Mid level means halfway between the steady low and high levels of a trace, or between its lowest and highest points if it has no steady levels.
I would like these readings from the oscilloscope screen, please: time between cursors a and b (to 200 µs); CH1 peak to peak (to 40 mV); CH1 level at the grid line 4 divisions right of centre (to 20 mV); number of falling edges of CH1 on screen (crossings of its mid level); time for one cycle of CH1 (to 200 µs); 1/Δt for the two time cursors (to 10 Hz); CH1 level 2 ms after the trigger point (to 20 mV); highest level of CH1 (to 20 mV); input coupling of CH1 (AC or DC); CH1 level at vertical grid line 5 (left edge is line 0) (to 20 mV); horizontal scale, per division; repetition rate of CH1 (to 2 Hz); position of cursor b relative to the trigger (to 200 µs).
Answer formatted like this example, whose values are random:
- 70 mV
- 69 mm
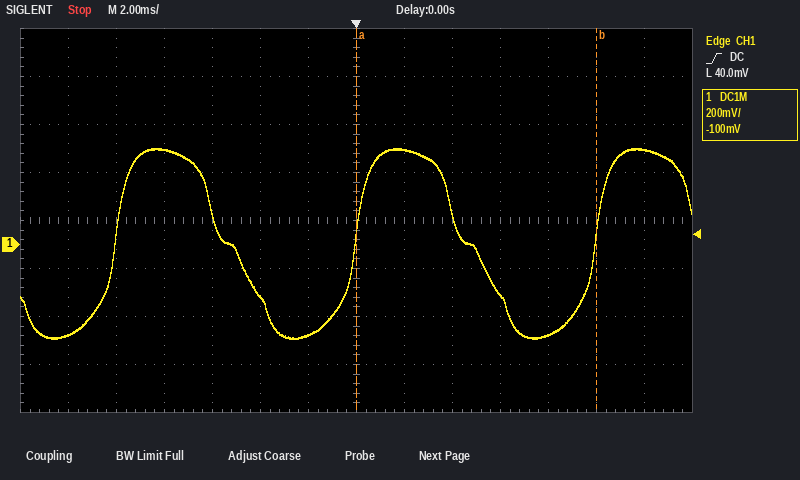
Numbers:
- 10.0 ms
- 800 mV
- -380 mV
- 2
- 10.0 ms
- 100 Hz
- 400 mV
- 400 mV
- DC
- -220 mV
- 2 ms
- 100 Hz
- +10.0 ms
